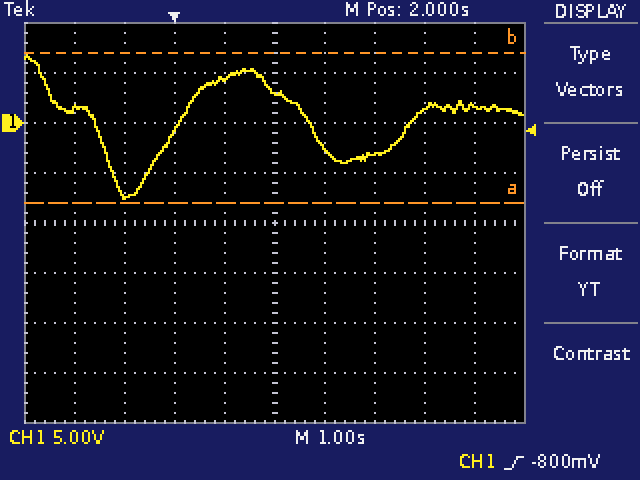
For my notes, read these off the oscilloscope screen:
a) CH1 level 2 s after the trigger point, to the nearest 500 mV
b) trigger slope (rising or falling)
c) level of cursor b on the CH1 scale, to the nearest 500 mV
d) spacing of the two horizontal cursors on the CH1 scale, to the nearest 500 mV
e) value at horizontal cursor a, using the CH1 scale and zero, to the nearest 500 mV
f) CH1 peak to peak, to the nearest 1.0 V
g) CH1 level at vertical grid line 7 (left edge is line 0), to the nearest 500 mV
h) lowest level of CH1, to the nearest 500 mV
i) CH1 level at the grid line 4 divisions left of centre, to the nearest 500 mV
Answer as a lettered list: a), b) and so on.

a) 3.0 V
b) rising
c) 7.0 V
d) 15.0 V
e) -8.0 V
f) 14.0 V
g) -3.0 V
h) -7.5 V
i) 1.5 V
